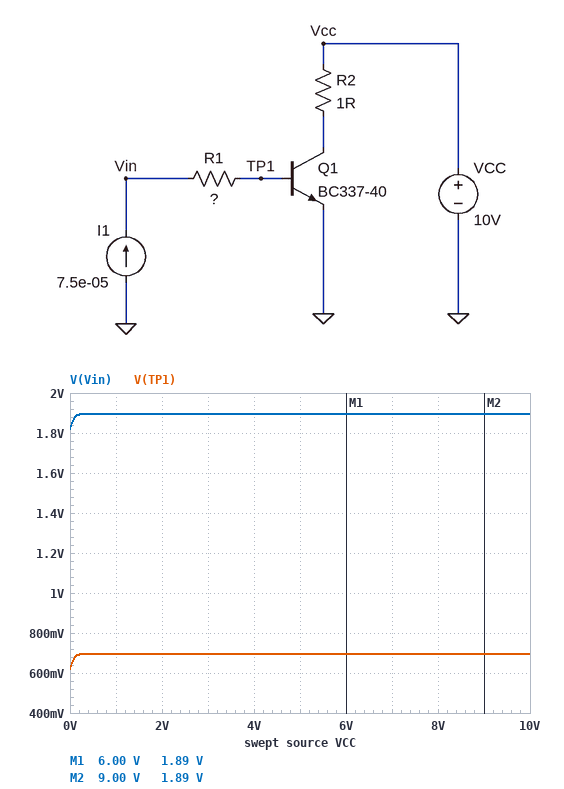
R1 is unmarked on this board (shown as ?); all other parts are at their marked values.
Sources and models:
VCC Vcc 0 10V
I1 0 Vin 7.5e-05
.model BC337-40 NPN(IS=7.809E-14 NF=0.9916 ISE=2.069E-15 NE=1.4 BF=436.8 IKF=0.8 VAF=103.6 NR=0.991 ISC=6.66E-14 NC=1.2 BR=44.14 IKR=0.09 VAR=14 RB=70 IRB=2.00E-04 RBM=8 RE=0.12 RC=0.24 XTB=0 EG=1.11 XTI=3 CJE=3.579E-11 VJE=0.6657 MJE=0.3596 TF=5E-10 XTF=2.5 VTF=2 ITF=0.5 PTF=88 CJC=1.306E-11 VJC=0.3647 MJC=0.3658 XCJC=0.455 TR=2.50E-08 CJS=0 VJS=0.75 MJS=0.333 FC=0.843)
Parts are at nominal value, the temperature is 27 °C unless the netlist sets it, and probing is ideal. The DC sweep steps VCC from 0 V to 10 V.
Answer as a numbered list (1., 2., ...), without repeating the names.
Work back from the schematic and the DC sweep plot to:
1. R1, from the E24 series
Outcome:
1. 16 kΩ
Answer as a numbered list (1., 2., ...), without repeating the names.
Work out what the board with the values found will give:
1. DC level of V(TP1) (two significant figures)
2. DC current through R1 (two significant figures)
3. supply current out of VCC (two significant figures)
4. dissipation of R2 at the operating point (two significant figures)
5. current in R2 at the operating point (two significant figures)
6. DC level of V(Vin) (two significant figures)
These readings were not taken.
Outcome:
1. 690 mV
2. 75 µA
3. 33 mA
4. 1.1 mW
5. 33 mA
6. 1.9 V
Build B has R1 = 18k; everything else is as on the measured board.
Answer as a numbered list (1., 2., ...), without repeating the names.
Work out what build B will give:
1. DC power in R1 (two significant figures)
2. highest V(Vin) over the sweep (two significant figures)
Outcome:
1. 100 µW
2. 2.0 V
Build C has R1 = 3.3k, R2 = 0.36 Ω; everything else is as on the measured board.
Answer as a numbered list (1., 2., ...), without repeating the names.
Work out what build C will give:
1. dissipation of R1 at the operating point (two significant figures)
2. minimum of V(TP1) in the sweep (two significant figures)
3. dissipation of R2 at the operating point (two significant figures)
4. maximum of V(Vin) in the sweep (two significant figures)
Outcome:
1. 19 µW
2. 620 mV
3. 380 µW
4. 940 mV
